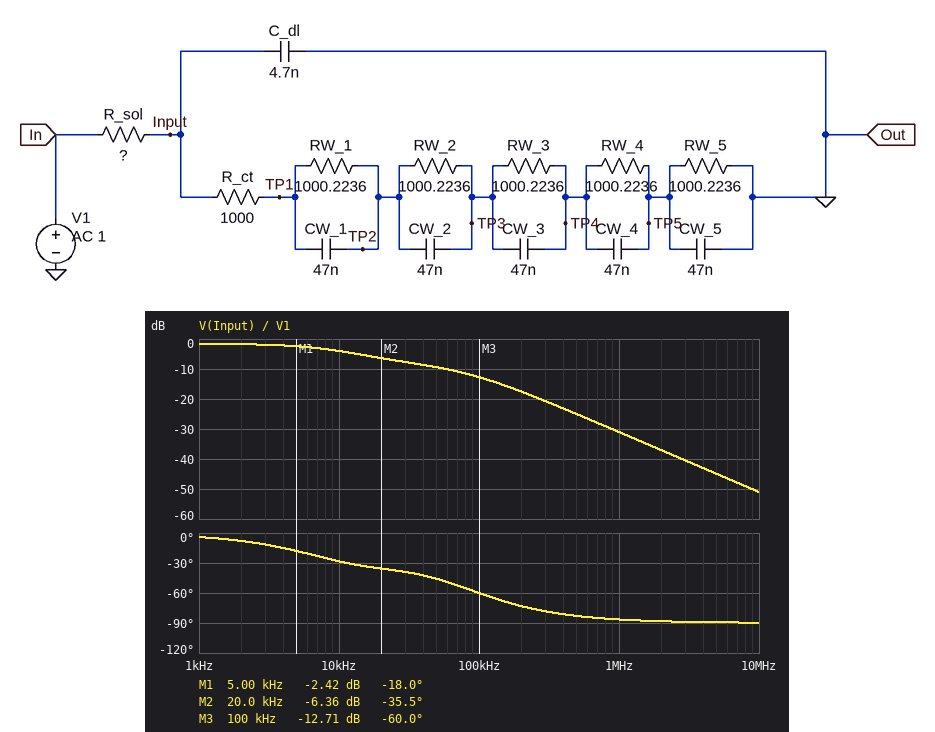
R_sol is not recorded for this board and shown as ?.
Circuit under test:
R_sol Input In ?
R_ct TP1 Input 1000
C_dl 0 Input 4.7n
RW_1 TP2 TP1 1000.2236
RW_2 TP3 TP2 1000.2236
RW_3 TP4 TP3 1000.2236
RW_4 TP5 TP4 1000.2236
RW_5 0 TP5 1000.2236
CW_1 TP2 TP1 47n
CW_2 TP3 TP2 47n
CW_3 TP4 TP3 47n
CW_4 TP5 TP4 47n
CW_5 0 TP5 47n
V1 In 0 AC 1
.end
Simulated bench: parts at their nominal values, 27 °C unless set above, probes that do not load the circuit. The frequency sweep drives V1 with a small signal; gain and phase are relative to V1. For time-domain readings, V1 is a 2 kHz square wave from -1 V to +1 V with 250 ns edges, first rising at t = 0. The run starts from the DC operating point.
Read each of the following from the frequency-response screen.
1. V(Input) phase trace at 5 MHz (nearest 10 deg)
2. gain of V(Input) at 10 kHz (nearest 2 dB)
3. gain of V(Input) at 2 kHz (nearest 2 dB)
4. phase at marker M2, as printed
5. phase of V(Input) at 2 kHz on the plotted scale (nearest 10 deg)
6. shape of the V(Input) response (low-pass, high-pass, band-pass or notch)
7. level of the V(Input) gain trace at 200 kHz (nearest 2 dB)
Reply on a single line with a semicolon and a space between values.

-90 deg; -4 dB; -2 dB; -35.5 deg; -10 deg; low-pass; -18 dB
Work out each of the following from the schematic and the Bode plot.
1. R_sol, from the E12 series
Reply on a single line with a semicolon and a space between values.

1.2 kΩ
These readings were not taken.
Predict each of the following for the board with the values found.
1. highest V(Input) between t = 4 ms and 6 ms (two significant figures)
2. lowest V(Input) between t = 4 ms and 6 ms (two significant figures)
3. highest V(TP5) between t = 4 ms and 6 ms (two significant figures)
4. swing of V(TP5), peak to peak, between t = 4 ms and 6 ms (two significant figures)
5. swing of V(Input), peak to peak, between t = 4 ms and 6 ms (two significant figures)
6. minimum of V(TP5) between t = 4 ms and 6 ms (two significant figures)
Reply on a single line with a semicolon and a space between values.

830 mV; -830 mV; 140 mV; 280 mV; 1.7 V; -140 mV
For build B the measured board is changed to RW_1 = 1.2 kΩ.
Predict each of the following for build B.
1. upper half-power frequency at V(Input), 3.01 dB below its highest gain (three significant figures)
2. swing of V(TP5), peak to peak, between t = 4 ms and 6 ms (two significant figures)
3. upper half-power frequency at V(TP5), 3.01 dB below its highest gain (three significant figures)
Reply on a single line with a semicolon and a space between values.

11.9 kHz; 270 mV; 9.81 kHz
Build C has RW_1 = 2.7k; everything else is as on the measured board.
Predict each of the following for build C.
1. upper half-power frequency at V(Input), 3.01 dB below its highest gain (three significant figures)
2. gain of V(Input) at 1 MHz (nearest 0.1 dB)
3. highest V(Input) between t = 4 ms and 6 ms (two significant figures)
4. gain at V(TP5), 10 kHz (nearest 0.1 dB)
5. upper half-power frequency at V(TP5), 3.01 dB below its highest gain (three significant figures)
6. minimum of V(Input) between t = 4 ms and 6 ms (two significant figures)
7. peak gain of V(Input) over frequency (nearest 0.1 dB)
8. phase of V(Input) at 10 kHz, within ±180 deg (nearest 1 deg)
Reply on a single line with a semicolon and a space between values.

10.9 kHz; -31.0 dB; 860 mV; -20.4 dB; 10.6 kHz; -860 mV; -1.3 dB; -29 deg
